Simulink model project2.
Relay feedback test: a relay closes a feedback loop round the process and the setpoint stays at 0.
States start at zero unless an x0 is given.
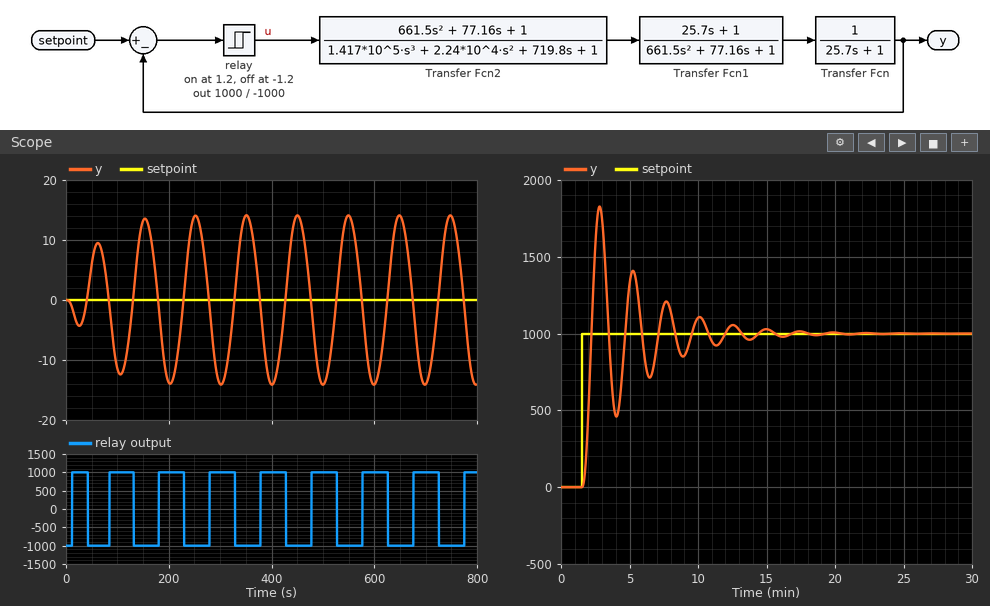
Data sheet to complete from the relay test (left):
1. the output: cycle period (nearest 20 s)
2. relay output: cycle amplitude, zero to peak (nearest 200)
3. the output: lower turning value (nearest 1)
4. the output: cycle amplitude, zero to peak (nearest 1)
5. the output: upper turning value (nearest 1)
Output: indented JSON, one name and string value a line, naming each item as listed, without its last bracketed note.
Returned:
{
  "the output: cycle period": "100 s",
  "relay output: cycle amplitude, zero to peak": "1000",
  "the output: lower turning value": "-14",
  "the output: cycle amplitude, zero to peak": "14",
  "the output: upper turning value": "14"
}
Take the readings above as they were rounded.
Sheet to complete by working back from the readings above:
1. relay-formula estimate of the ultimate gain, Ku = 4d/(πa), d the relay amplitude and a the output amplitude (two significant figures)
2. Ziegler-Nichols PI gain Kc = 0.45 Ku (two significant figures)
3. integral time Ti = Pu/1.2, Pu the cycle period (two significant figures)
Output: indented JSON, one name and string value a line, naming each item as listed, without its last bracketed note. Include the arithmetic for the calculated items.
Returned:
{
  "relay-formula estimate of the ultimate gain, Ku = 4d/(πa), d the relay amplitude and a the output amplitude": "4 × 1000 / (π × 14) = 91",
  "Ziegler-Nichols PI gain Kc = 0.45 Ku": "0.45 × 91 = 41",
  "integral time Ti = Pu/1.2, Pu the cycle period": "100 / 1.2 = 83 s"
}
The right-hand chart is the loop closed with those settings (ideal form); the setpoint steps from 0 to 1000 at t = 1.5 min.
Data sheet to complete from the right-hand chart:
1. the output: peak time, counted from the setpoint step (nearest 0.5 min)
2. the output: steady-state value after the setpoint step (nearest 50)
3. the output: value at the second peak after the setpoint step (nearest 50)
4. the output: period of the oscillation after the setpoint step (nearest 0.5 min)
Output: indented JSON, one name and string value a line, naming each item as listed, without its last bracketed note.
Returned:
{
  "the output: peak time, counted from the setpoint step": "1.5 min",
  "the output: steady-state value after the setpoint step": "1000",
  "the output: value at the second peak after the setpoint step": "1400",
  "the output: period of the oscillation after the setpoint step": "2.5 min"
}
